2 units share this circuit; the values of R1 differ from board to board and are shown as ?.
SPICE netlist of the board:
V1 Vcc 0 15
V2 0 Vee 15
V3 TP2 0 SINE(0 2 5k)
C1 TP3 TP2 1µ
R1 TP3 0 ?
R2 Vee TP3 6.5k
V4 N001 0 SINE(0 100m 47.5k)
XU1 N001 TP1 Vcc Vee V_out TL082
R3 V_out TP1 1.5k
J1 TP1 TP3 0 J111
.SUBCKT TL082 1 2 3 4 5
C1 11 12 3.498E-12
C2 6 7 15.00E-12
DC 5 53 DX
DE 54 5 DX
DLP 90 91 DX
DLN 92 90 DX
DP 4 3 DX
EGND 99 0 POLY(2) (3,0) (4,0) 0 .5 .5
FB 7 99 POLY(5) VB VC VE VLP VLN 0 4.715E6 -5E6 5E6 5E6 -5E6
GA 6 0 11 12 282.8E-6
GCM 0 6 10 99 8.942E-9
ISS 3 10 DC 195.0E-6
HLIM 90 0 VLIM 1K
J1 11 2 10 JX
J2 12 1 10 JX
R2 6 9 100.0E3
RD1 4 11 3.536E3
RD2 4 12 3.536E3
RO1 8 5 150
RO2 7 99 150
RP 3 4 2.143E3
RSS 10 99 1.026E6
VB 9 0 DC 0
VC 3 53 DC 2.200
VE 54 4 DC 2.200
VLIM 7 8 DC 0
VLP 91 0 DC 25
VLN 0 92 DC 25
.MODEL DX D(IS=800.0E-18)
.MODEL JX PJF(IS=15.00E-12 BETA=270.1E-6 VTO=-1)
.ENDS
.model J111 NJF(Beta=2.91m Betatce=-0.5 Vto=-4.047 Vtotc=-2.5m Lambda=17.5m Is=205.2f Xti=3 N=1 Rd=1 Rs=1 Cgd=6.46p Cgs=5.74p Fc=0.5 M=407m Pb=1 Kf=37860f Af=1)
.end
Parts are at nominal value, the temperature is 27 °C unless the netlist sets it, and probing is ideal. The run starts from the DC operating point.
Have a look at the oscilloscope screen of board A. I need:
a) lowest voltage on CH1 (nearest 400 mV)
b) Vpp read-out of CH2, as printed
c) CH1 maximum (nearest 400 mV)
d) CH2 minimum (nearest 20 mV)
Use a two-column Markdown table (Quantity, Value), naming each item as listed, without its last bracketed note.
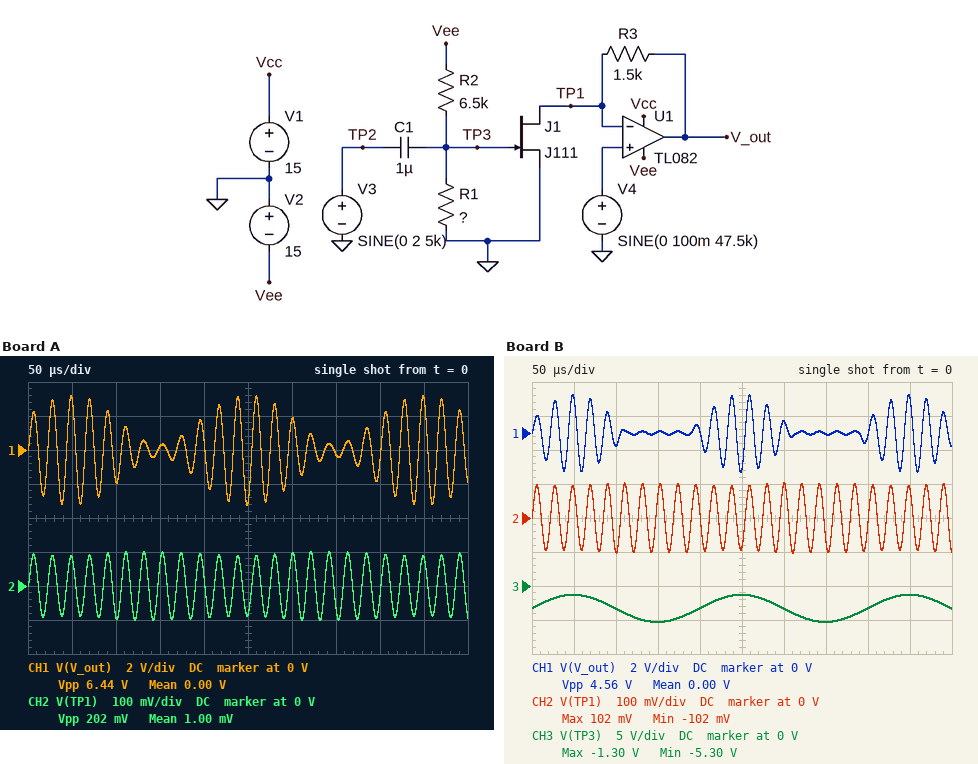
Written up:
| Quantity | Value |
|---|---|
| lowest voltage on CH1 | -3.2 V |
| Vpp read-out of CH2, as printed | 202 mV |
| CH1 maximum | 3.2 V |
| CH2 minimum | -100 mV |
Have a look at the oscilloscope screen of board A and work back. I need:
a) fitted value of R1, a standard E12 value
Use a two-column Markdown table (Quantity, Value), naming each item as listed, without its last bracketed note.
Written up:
| Quantity | Value |
|---|---|
| fitted value of R1, a standard E12 value | 820 Ω |
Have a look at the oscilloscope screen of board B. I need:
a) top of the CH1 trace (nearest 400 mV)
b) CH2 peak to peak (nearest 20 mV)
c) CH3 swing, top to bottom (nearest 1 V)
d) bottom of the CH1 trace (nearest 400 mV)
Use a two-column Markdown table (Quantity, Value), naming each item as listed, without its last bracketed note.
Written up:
| Quantity | Value |
|---|---|
| top of the CH1 trace | 2.4 V |
| CH2 peak to peak | 200 mV |
| CH3 swing, top to bottom | 4 V |
| bottom of the CH1 trace | -2.4 V |
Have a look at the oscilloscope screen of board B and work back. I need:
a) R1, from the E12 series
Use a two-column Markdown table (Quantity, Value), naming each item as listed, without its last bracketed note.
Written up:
| Quantity | Value |
|---|---|
| R1, from the E12 series | 1.8 kΩ |
